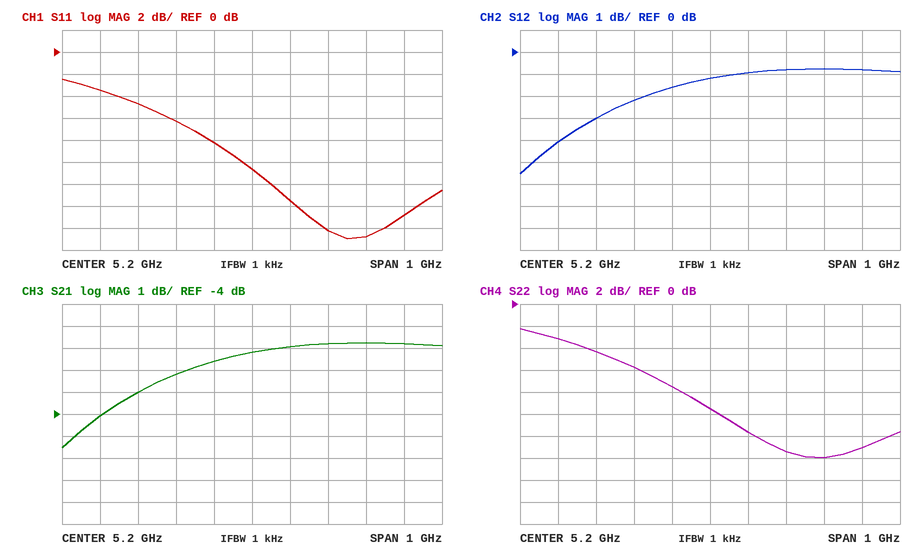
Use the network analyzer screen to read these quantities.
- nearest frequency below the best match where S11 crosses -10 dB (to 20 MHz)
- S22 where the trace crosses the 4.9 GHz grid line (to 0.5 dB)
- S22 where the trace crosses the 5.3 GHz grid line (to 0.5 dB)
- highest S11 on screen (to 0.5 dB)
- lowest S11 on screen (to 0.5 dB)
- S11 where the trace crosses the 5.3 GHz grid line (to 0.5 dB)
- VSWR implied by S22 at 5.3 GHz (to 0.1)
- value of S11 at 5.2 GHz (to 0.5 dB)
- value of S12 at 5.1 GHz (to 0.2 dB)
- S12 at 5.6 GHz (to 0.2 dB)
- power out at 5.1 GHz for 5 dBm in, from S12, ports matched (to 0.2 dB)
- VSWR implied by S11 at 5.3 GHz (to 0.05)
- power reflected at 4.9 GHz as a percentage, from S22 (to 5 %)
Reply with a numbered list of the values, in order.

1. 5.18 GHz
2. -4.5 dB
3. -11.5 dB
4. -2.5 dB
5. -17.0 dB
6. -13.5 dB
7. 1.7
8. -10.5 dB
9. -1.6 dB
10. -0.8 dB
11. 3.4 dBm
12. 1.55
13. 35 %
